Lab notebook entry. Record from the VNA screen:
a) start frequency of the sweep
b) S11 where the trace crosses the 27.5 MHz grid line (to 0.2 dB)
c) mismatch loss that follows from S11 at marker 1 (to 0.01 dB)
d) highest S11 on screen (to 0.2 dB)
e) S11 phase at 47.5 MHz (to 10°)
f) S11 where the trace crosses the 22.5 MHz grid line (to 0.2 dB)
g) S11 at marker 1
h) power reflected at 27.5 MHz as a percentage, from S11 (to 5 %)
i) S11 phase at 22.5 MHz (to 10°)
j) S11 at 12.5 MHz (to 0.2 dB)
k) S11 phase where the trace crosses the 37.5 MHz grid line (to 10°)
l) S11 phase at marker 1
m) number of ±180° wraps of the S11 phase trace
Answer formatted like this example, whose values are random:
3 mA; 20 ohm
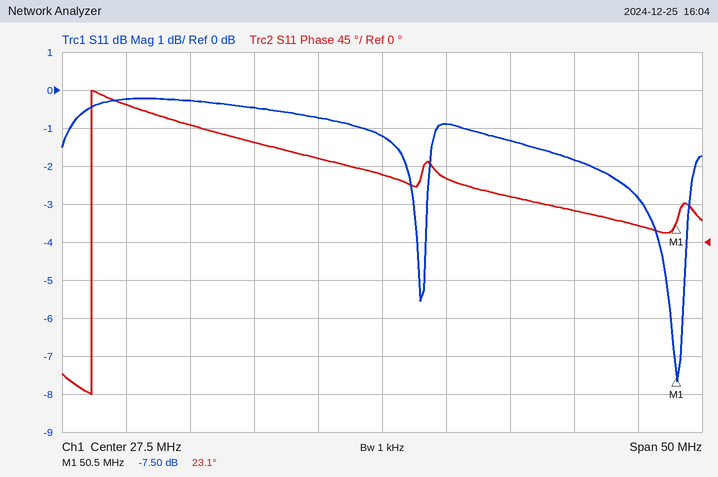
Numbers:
2.5 MHz; -1.2 dB; 0.85 dB; -0.2 dB; 20°; -0.8 dB; -7.50 dB; 75 %; 100°; -0.2 dB; 50°; 23.1°; 1
